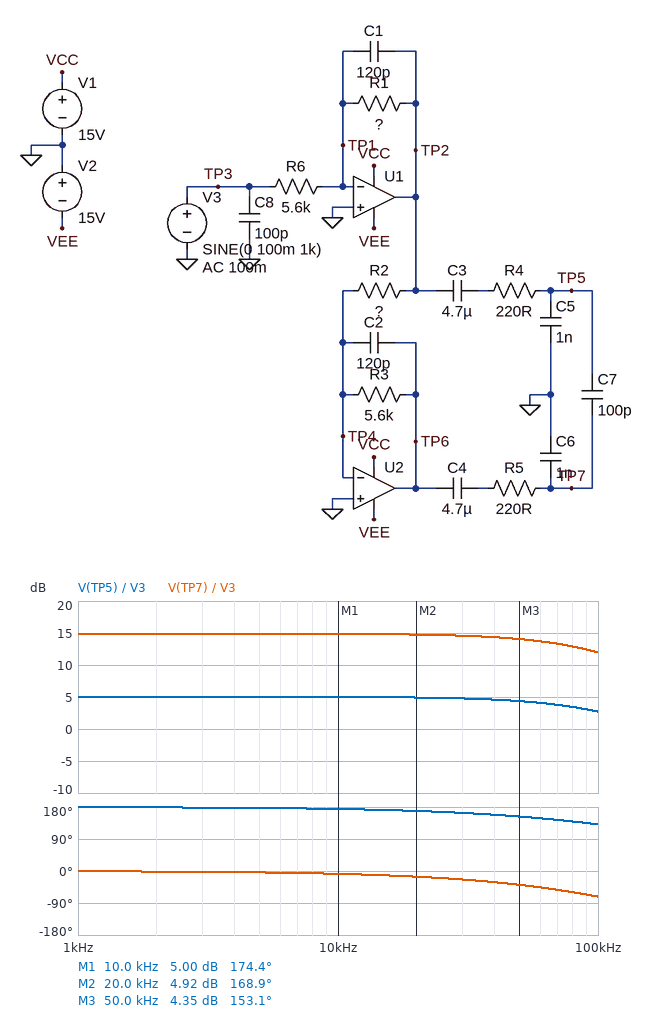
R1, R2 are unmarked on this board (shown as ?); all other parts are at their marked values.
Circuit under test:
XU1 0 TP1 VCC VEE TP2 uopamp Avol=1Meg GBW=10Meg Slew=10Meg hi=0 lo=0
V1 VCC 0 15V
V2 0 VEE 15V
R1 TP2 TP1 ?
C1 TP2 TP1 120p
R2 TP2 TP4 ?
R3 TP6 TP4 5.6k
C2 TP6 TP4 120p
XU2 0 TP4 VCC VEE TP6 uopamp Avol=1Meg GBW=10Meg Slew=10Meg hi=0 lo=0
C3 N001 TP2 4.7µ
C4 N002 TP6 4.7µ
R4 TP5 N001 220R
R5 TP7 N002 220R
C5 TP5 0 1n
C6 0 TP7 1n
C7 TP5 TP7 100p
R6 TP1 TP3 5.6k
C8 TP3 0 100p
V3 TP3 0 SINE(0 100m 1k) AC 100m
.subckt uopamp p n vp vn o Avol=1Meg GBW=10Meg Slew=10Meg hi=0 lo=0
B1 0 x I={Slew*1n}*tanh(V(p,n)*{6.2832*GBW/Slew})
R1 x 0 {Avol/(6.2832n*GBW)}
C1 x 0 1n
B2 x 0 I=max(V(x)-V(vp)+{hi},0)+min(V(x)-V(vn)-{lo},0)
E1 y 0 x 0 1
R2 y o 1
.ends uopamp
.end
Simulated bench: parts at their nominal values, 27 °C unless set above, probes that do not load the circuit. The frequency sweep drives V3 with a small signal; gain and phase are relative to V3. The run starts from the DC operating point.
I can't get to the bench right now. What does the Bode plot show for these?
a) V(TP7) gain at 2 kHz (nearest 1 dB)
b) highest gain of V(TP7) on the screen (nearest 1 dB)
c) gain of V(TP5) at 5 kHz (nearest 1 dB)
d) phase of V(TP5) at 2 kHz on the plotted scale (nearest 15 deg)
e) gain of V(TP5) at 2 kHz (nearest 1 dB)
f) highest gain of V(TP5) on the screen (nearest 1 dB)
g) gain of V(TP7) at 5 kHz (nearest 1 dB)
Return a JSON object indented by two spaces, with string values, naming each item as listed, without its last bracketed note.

{
  "V(TP7) gain at 2 kHz": "15 dB",
  "highest gain of V(TP7) on the screen": "15 dB",
  "gain of V(TP5) at 5 kHz": "5 dB",
  "phase of V(TP5) at 2 kHz on the plotted scale": "180 deg",
  "gain of V(TP5) at 2 kHz": "5 dB",
  "highest gain of V(TP5) on the screen": "5 dB",
  "gain of V(TP7) at 5 kHz": "15 dB"
}
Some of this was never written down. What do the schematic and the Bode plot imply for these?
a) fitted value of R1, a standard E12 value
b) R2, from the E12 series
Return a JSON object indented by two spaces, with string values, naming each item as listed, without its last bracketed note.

{
  "fitted value of R1, a standard E12 value": "10 kΩ",
  "R2, from the E12 series": "1.8 kΩ"
}
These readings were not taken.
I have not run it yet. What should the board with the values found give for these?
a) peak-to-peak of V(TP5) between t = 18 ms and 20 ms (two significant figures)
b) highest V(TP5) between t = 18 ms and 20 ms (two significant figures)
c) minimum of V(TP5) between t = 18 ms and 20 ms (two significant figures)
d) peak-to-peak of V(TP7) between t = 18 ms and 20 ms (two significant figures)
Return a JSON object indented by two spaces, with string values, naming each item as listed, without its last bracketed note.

{
  "peak-to-peak of V(TP5) between t = 18 ms and 20 ms": "360 mV",
  "highest V(TP5) between t = 18 ms and 20 ms": "180 mV",
  "minimum of V(TP5) between t = 18 ms and 20 ms": "-180 mV",
  "peak-to-peak of V(TP7) between t = 18 ms and 20 ms": "1.1 V"
}
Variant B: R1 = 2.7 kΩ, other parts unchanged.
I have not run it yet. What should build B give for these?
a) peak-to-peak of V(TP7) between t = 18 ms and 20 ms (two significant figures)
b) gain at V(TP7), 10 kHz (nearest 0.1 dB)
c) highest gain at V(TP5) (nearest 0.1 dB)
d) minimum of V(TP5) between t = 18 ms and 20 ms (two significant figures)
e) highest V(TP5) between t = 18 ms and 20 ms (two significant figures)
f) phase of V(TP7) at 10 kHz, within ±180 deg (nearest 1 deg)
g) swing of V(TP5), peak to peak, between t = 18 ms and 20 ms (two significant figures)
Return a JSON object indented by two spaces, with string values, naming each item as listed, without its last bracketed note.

{
  "peak-to-peak of V(TP7) between t = 18 ms and 20 ms": "300 mV",
  "gain at V(TP7), 10 kHz": "3.5 dB",
  "highest gain at V(TP5)": "-6.3 dB",
  "minimum of V(TP5) between t = 18 ms and 20 ms": "-48 mV",
  "highest V(TP5) between t = 18 ms and 20 ms": "48 mV",
  "phase of V(TP7) at 10 kHz, within ±180 deg": "-5 deg",
  "swing of V(TP5), peak to peak, between t = 18 ms and 20 ms": "96 mV"
}
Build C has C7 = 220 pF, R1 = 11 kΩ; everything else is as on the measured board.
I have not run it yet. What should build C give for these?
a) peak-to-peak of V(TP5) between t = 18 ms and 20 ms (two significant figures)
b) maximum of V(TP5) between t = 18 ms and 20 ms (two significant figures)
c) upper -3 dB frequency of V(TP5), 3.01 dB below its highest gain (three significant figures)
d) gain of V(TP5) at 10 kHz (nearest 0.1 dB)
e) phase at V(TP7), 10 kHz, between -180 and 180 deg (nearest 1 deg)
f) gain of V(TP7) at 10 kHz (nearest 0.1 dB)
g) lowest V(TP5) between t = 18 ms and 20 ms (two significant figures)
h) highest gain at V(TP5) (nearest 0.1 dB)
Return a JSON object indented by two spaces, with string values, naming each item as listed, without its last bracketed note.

{
  "peak-to-peak of V(TP5) between t = 18 ms and 20 ms": "390 mV",
  "maximum of V(TP5) between t = 18 ms and 20 ms": "200 mV",
  "upper -3 dB frequency of V(TP5), 3.01 dB below its highest gain": "103 kHz",
  "gain of V(TP5) at 10 kHz": "5.8 dB",
  "phase at V(TP7), 10 kHz, between -180 and 180 deg": "-9 deg",
  "gain of V(TP7) at 10 kHz": "15.7 dB",
  "lowest V(TP5) between t = 18 ms and 20 ms": "-200 mV",
  "highest gain at V(TP5)": "5.9 dB"
}
